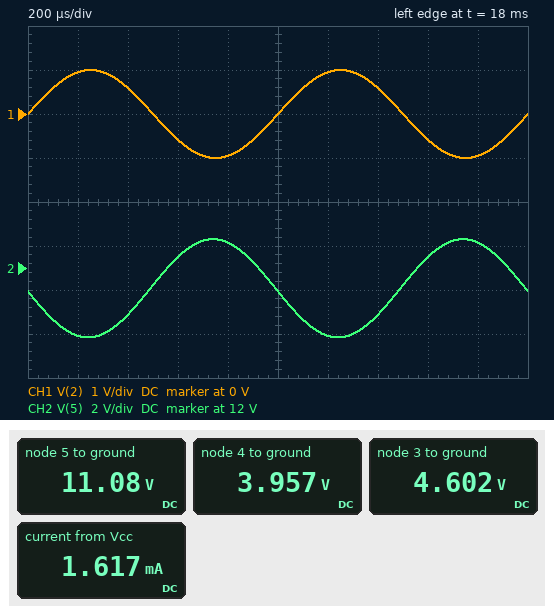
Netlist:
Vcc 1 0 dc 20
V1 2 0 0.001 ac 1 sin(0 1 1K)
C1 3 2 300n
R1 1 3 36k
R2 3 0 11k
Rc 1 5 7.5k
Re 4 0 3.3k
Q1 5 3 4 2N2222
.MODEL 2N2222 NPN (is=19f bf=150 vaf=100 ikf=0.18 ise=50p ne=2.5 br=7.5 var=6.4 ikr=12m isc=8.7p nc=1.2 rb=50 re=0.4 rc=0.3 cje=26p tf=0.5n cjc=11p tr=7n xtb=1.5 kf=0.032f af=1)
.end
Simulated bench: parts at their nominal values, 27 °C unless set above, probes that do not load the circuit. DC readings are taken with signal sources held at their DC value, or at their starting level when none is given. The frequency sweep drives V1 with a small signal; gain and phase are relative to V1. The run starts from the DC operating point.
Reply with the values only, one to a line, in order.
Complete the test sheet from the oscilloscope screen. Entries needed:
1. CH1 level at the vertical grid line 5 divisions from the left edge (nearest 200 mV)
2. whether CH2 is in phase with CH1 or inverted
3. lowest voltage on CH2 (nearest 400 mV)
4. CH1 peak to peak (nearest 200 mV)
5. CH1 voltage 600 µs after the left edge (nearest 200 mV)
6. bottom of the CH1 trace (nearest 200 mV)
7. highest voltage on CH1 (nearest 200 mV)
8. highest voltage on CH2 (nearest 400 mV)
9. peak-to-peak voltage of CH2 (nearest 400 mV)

0 V
inverted
8.8 V
2.0 V
-600 mV
-1.0 V
1.0 V
13.2 V
4.4 V
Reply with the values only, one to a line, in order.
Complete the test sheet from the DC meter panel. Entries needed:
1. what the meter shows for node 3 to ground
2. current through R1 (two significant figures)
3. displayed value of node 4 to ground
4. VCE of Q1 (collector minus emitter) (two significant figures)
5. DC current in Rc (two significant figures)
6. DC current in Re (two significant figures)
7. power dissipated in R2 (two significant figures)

4.602 V
430 µA
3.957 V
7.1 V
1.2 mA
1.2 mA
1.9 mW
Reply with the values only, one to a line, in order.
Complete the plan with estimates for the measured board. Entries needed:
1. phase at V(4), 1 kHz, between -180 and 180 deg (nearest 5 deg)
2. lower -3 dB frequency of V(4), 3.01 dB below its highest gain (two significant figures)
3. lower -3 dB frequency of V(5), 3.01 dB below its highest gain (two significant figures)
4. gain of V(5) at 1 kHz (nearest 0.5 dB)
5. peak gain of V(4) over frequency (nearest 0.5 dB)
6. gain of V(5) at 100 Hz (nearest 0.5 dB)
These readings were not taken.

5 deg
64 Hz
64 Hz
7.0 dB
0 dB
5.5 dB
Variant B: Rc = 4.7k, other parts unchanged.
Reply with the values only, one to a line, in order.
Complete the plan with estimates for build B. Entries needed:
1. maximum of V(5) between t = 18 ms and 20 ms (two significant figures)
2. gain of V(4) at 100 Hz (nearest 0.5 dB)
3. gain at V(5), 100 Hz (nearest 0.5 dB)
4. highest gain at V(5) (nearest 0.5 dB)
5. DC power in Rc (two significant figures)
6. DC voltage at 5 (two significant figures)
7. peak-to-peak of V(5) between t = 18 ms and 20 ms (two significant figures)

16 V
-1.5 dB
1.5 dB
3.0 dB
6.7 mW
14 V
2.8 V
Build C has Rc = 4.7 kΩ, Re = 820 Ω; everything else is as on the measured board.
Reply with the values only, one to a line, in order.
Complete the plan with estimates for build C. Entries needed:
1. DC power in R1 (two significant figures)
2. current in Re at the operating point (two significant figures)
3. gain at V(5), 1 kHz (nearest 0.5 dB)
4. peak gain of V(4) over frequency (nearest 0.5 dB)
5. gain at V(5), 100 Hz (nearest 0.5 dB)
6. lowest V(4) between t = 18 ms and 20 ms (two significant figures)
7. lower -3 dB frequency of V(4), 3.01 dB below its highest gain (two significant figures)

7.4 mW
3.7 mA
-8.0 dB
-0.5 dB
-23.5 dB
1.6 V
720 Hz
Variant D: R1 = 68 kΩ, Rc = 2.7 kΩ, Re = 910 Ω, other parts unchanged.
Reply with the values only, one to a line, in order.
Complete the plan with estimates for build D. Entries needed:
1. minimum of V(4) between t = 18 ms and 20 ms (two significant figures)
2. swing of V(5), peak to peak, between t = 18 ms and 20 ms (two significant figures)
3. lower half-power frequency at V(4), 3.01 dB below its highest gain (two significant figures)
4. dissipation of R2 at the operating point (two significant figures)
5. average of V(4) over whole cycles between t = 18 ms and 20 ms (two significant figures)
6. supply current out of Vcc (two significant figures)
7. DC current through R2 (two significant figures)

1.0 V
5.8 V
60 Hz
630 µW
2.0 V
2.4 mA
240 µA
